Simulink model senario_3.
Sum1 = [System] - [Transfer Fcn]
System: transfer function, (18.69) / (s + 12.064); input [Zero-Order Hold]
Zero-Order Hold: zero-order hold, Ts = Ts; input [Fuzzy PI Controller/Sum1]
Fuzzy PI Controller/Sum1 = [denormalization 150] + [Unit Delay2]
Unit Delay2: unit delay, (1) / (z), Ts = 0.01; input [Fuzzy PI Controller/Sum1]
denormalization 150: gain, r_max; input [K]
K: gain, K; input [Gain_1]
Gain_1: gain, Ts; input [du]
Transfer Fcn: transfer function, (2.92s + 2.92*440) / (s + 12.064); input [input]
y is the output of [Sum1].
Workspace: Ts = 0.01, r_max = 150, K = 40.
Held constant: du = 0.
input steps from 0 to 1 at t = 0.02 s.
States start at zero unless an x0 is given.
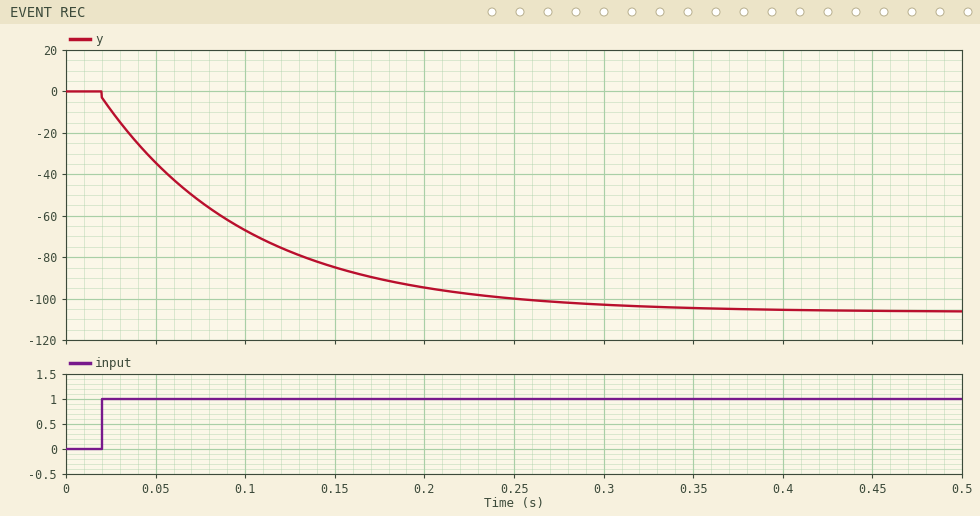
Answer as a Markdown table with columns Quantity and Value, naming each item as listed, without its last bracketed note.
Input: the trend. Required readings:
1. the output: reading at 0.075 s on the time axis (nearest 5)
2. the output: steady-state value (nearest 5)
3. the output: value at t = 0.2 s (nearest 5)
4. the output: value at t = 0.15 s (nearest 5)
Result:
| Quantity | Value |
|---|---|
| the output: reading at 0.075 s on the time axis | -55 |
| the output: steady-state value | -105 |
| the output: value at t = 0.2 s | -95 |
| the output: value at t = 0.15 s | -85 |
